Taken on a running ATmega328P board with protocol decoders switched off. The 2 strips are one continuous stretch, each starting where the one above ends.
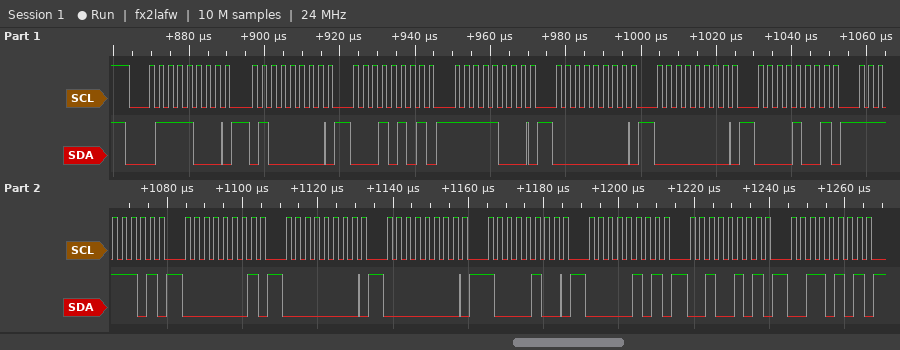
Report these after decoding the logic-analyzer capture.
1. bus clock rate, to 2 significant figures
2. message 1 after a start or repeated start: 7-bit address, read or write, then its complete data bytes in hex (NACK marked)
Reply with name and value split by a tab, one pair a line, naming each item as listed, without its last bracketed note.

bus clock rate, to 2 significant figures	400 kHz
message 1 after a start or repeated start: 7-bit address, read or write, then its complete data bytes in hex	0x3C write: 40 15 F8 00 00 09 FD 01 00 00 84 05 25 35
